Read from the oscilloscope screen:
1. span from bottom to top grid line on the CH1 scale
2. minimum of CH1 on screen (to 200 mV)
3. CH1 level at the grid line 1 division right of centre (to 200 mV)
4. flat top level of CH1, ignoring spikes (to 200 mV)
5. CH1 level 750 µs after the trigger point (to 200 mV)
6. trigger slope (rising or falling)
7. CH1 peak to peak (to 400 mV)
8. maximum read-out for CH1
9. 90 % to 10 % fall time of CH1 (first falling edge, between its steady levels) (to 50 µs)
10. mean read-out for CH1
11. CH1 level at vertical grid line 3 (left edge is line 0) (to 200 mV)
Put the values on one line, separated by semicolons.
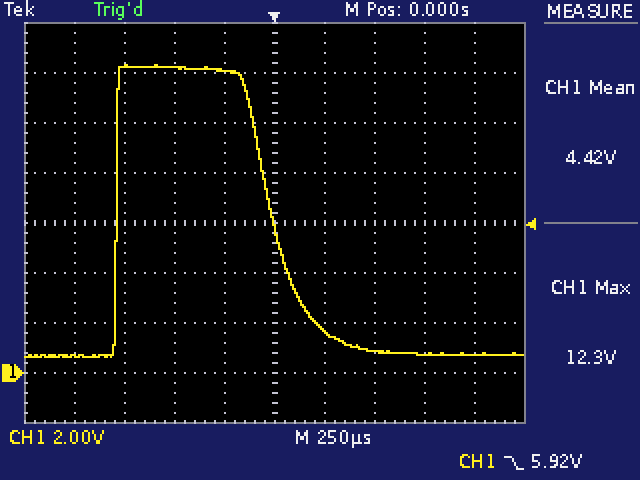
16 V; 600 mV; 1.6 V; 12.2 V; 800 mV; falling; 11.6 V; 12.3 V; 350 µs; 4.42 V; 12.2 V
